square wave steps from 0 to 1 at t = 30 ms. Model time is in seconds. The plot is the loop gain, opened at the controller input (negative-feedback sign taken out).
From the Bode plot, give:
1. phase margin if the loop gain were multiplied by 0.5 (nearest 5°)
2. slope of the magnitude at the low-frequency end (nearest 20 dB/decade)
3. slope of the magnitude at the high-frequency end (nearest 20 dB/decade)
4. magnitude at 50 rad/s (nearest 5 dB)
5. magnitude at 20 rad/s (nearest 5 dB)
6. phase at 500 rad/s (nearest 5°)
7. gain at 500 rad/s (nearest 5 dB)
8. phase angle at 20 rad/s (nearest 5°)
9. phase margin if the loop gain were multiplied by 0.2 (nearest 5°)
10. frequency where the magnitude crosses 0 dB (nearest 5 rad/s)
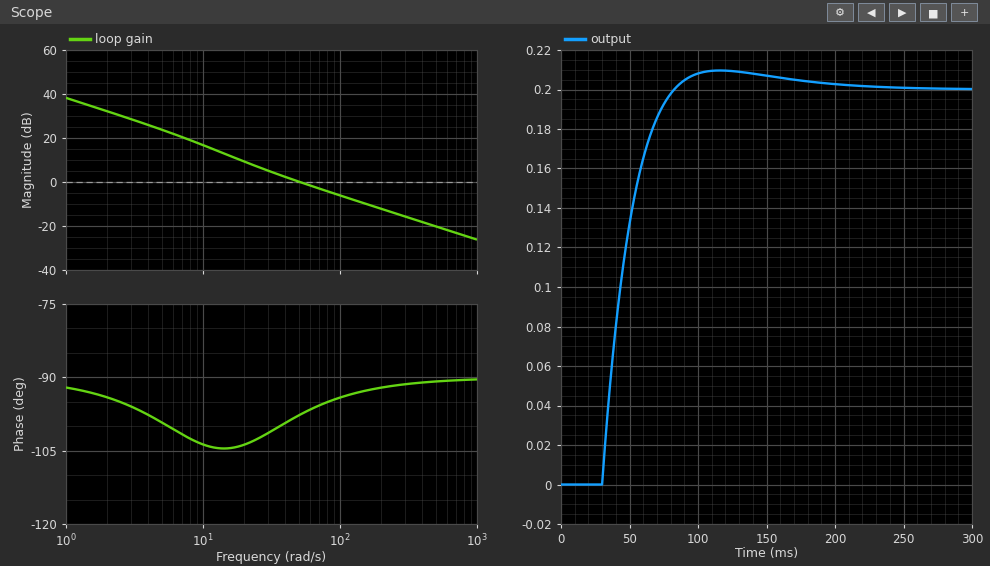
80°
-20 dB/decade
-20 dB/decade
0 dB
10 dB
-90°
-20 dB
-105°
75°
50 rad/s
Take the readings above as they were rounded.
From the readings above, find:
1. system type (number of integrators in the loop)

1
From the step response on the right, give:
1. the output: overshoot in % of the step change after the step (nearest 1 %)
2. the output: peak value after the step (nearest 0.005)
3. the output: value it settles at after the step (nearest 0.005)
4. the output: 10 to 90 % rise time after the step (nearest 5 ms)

5 %
0.210
0.200
35 ms
